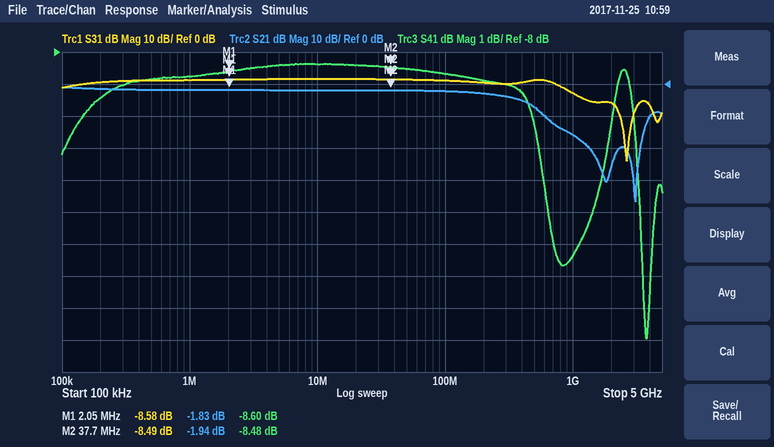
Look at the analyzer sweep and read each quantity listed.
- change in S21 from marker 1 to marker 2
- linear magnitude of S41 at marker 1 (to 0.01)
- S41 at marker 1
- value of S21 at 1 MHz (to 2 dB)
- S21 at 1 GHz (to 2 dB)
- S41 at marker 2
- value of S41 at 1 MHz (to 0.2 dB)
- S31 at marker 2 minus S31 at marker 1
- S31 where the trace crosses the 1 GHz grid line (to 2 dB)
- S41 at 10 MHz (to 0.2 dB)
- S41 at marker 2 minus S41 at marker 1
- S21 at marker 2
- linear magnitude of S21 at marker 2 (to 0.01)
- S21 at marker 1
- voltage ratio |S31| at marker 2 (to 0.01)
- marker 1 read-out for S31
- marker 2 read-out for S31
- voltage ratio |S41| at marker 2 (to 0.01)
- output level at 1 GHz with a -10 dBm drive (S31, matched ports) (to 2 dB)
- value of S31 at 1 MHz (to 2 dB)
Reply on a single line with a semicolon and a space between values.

-0.11 dB; 0.37; -8.60 dB; -2 dB; -16 dB; -8.48 dB; -8.8 dB; 0.09 dB; -12 dB; -8.4 dB; 0.12 dB; -1.94 dB; 0.80; -1.83 dB; 0.38; -8.58 dB; -8.49 dB; 0.38; -22 dBm; -8 dB
